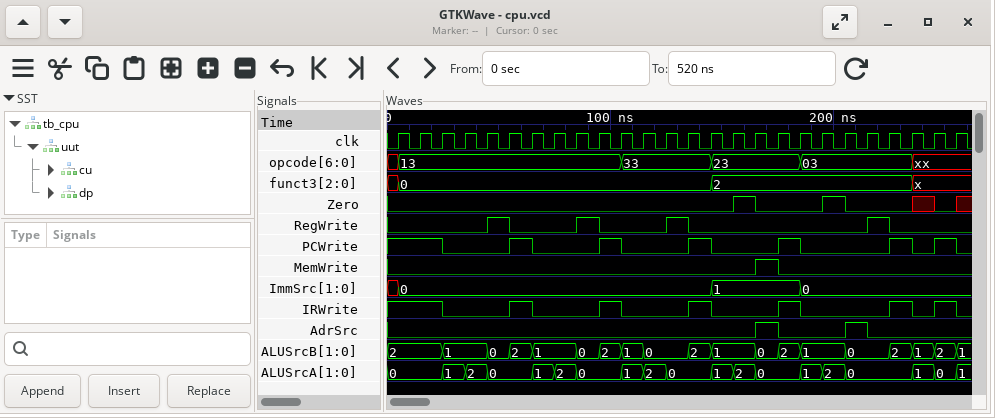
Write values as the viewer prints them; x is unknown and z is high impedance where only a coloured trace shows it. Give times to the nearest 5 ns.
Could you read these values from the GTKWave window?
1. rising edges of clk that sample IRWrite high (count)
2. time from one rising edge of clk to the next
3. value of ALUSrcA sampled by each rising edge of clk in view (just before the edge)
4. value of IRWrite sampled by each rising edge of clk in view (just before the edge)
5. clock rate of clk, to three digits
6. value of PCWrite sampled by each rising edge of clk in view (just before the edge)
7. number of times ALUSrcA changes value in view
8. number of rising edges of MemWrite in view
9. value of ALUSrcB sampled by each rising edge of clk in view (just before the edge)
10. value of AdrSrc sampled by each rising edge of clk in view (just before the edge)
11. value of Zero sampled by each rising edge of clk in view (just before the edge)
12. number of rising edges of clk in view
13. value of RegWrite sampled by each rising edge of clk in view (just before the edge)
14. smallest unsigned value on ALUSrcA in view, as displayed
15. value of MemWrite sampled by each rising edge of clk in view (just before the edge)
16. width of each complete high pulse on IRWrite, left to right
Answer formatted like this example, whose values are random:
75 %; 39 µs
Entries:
9; 10 ns; 0, 0, 0, 1, 2, 0, 0, 1, 2, 0, 0, 1, 2, 0, 0, 1, 2, 0, 0, 1, 2, 0, 0, 0, 1, 0; 1 1 1 0 0 0 1 0 0 0 1 0 0 0 1 0 0 0 1 0 0 0 0 1 0 1; 100 MHz; 1 1 1 0 0 0 1 0 0 0 1 0 0 0 1 0 0 0 1 0 0 0 0 1 0 1; 18; 1; 2, 2, 2, 1, 1, 0, 2, 1, 1, 0, 2, 1, 0, 0, 2, 1, 1, 0, 2, 1, 1, 0, 0, 2, 1, 2; 0 0 0 0 0 0 0 0 0 0 0 0 0 0 0 0 0 1 0 0 0 1 0 0 0 0; 0 0 0 0 0 0 0 0 0 0 0 0 0 0 0 0 1 0 0 0 1 0 0 0 x 0; 26; 0 0 0 0 0 1 0 0 0 1 0 0 0 1 0 0 0 0 0 0 0 0 1 0 0 0; 0; 0 0 0 0 0 0 0 0 0 0 0 0 0 0 0 0 0 1 0 0 0 0 0 0 0 0; 10 ns, 10 ns, 10 ns, 10 ns, 10 ns, 10 ns
